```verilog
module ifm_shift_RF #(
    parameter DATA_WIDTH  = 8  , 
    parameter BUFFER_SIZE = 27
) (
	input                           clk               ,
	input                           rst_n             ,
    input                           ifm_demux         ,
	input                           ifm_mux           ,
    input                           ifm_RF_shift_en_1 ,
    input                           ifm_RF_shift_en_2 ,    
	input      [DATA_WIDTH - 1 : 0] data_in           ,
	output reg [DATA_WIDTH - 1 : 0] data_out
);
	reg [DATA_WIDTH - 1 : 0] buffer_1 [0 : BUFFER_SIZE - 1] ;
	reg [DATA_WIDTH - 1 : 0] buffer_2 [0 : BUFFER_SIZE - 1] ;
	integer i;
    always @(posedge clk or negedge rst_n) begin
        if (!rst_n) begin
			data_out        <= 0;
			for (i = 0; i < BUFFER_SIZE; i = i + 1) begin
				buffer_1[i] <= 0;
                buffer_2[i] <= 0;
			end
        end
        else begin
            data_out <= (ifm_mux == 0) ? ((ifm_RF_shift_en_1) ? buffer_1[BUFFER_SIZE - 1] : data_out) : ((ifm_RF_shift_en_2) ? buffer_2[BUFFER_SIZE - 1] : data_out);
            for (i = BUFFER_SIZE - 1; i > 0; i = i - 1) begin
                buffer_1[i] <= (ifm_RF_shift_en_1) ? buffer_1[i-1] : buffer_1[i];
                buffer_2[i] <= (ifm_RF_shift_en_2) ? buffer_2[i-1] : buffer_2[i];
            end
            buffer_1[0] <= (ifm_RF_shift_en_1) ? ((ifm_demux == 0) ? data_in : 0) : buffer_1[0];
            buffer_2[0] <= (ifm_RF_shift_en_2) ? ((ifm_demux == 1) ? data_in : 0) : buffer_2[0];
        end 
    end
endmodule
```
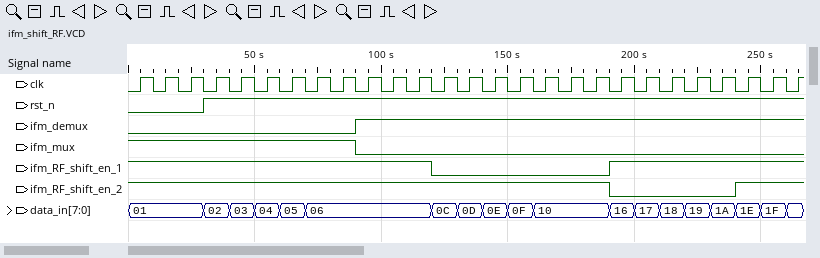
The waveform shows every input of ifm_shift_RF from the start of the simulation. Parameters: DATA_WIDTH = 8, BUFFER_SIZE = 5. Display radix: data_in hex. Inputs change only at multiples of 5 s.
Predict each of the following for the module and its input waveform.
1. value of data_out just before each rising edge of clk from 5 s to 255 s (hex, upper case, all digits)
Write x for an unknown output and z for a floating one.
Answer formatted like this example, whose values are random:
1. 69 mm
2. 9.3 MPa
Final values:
1. 00, 00, 00, 00, 00, 00, 00, 00, 00, 00, 03, 04, 05, 05, 05, 05, 05, 05, 05, 05, 06, 06, 00, 00, 00, 00
